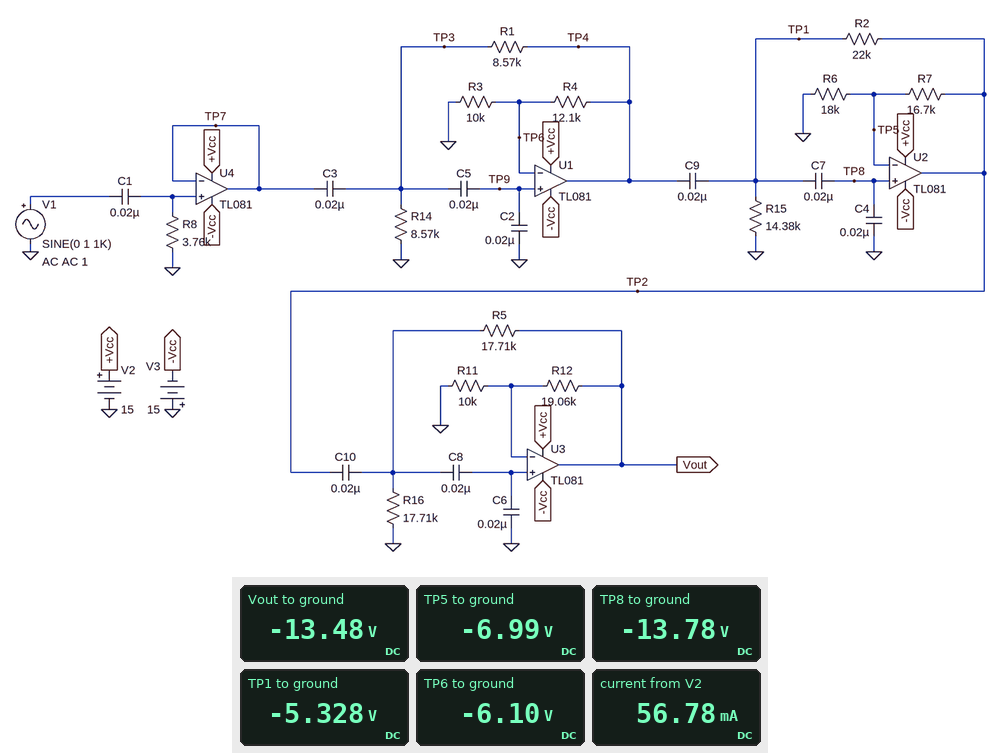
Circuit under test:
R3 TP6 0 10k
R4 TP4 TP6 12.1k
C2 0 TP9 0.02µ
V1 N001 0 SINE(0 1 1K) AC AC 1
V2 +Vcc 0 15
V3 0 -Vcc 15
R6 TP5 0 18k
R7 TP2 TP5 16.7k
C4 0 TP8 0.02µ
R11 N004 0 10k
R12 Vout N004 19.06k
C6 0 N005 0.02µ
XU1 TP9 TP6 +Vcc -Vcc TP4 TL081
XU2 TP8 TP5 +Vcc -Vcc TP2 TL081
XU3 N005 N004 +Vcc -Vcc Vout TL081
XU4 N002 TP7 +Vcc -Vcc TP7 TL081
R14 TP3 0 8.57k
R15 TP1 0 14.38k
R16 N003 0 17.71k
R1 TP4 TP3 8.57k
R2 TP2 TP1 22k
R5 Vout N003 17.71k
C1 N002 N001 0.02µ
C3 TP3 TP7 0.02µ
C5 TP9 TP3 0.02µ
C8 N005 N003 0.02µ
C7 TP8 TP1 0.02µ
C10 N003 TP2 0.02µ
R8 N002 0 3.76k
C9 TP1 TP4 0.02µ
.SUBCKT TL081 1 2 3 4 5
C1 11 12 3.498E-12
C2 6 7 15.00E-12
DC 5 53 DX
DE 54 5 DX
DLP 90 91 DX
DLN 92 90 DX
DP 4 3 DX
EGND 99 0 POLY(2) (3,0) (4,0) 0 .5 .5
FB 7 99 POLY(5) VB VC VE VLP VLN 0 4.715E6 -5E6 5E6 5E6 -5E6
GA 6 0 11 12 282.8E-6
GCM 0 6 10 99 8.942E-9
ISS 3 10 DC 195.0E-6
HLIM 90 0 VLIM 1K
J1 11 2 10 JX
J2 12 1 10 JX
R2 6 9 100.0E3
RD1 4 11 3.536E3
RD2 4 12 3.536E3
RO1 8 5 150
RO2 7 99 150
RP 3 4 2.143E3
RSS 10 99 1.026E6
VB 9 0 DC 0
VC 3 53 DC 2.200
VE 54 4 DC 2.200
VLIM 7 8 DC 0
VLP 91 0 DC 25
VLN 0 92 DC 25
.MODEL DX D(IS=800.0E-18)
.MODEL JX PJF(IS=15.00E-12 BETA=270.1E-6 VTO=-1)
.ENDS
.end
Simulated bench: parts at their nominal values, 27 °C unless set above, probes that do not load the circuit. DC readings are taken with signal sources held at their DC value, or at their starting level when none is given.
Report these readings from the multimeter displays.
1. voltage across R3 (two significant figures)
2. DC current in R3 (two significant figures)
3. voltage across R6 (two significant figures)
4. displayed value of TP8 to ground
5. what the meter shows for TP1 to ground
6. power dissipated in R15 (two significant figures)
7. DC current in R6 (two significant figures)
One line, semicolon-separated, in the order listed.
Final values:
6.1 V; 610 µA; 7.0 V; -13.78 V; -5.328 V; 2.0 mW; 390 µA
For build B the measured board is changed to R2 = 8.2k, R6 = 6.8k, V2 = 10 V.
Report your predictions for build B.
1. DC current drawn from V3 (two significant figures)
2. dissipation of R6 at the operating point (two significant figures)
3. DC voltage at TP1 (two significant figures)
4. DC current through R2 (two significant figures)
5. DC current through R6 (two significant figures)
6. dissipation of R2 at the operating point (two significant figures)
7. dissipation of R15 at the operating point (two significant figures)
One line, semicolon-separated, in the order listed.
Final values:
47 mA; 2.2 mW; -8.6 V; 600 µA; 570 µA; 2.9 mW; 5.1 mW
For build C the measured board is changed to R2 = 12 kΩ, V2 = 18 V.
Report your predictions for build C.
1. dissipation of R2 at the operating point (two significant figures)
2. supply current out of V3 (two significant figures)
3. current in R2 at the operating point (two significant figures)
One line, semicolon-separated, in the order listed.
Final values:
3.1 mW; 62 mA; 510 µA
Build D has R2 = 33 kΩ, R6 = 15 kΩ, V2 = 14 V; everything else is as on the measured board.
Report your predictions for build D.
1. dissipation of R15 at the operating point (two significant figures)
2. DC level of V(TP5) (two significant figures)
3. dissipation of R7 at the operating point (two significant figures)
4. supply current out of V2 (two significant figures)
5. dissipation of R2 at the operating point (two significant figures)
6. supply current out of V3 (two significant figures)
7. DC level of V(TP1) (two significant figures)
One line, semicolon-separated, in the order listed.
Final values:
1.2 mW; -6.4 V; 3.0 mW; 55 mA; 2.7 mW; 54 mA; -4.1 V
